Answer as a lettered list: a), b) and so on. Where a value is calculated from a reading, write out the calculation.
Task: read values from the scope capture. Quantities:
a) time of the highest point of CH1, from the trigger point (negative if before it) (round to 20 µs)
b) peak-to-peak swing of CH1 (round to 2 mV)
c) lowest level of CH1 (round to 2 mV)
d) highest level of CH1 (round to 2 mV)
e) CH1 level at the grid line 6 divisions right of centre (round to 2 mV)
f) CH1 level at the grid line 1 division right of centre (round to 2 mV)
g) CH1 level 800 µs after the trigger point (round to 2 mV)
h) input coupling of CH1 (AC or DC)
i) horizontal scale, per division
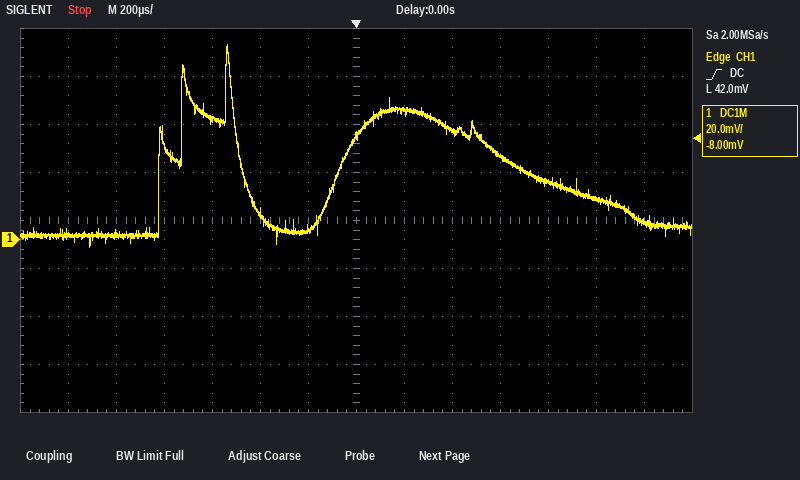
a) -540 µs
b) 82 mV − (-2 mV) = 84 mV
c) -2 mV
d) 82 mV
e) 8 mV
f) 54 mV
g) 24 mV
h) DC
i) 200 µs
